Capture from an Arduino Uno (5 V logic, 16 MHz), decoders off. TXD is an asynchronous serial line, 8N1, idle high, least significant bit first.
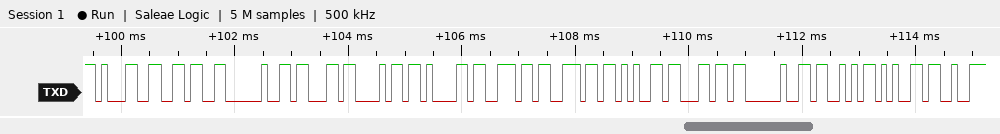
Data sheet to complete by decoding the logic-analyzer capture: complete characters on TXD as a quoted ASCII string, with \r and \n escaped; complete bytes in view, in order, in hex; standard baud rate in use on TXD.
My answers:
"16 channel Se"
31 36 20 63 68 61 6E 6E 65 6C 20 53 65
9600 baud
